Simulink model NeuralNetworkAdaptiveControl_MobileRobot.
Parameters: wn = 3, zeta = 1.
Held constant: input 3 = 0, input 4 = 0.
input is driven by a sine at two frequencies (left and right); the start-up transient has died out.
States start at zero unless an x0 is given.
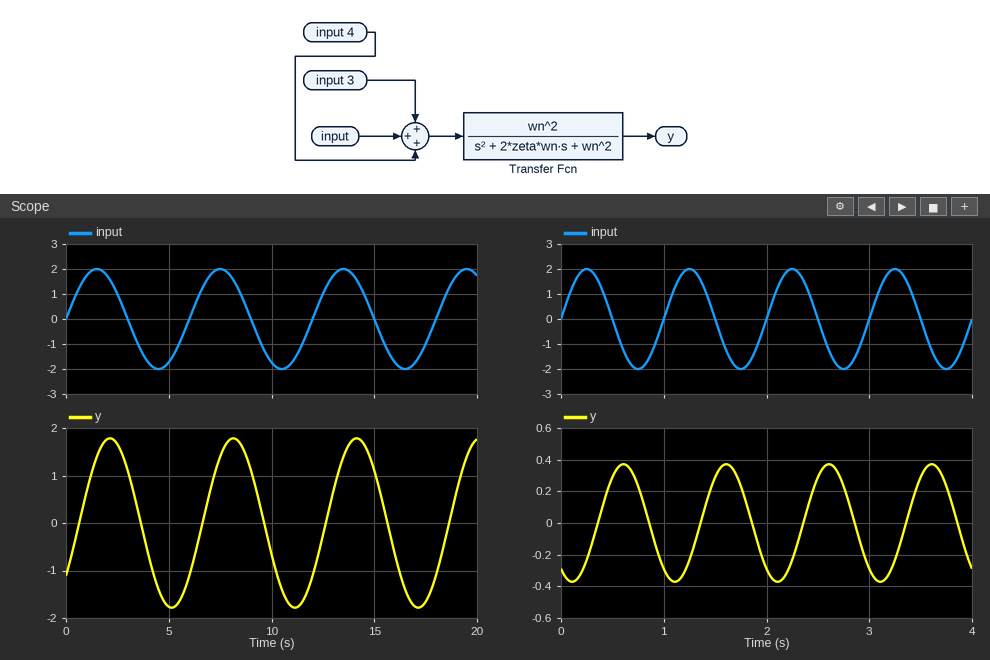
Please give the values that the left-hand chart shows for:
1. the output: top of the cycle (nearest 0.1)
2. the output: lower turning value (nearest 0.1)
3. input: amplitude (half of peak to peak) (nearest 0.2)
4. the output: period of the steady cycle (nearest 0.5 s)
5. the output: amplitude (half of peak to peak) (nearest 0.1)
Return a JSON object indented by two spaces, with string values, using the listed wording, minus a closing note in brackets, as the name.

{
  "the output: top of the cycle": "1.8",
  "the output: lower turning value": "-1.8",
  "input: amplitude (half of peak to peak)": "2.0",
  "the output: period of the steady cycle": "6.0 s",
  "the output: amplitude (half of peak to peak)": "1.8"
}
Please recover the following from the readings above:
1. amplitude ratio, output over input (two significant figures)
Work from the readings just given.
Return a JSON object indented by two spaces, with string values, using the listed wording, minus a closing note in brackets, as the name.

{
  "amplitude ratio, output over input": "0.90"
}
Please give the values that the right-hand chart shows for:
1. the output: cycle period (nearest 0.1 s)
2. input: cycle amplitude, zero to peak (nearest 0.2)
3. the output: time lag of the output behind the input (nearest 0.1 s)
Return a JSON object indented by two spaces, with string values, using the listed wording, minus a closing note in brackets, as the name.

{
  "the output: cycle period": "1.0 s",
  "input: cycle amplitude, zero to peak": "2.0",
  "the output: time lag of the output behind the input": "0.4 s"
}
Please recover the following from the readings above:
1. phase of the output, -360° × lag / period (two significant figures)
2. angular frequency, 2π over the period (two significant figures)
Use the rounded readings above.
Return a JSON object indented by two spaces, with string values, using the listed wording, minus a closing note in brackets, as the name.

{
  "phase of the output, -360° × lag / period": "-140°",
  "angular frequency, 2π over the period": "6.3 rad/s"
}
